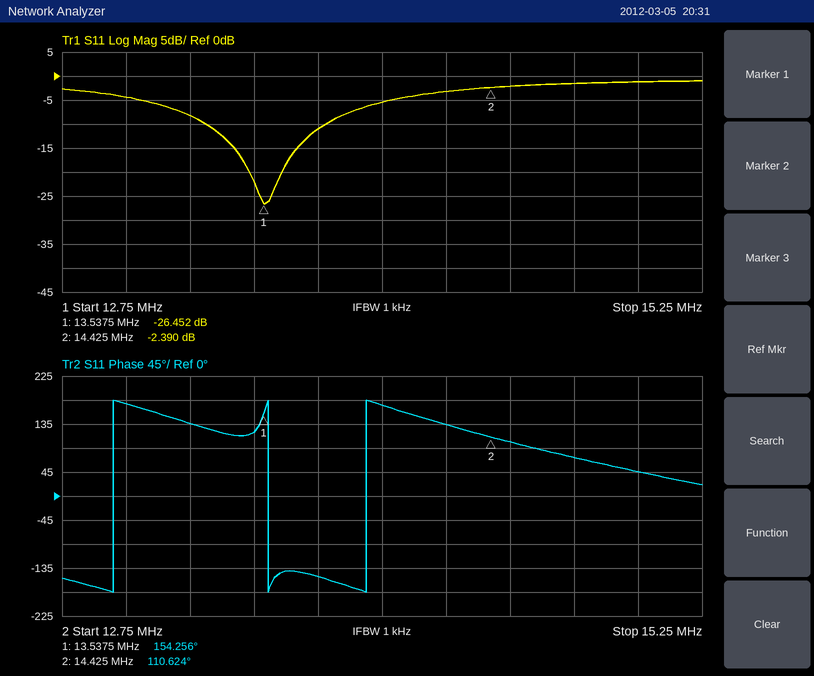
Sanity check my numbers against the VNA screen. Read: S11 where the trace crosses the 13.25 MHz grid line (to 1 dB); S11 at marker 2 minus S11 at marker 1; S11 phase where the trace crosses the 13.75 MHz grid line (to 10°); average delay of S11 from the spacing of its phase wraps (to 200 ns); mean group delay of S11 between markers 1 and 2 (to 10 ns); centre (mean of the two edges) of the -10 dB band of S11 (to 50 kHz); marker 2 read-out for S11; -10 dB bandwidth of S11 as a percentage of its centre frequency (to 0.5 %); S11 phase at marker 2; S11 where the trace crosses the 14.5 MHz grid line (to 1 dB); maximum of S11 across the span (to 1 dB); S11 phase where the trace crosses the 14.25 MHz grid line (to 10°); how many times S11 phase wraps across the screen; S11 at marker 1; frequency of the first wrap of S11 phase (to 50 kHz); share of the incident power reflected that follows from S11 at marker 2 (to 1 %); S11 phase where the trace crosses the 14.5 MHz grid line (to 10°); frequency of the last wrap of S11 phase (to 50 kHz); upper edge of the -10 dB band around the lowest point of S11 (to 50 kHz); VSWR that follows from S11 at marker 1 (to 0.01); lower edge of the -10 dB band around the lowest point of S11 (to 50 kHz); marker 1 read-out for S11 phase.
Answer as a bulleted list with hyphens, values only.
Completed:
- -8 dB
- 24.062 dB
- -150°
- 2.0 µs
- 140 ns
- 13.55 MHz
- -2.390 dB
- 3.5 %
- 110.624°
- -2 dB
- -1 dB
- 130°
- 3
- -26.452 dB
- 12.95 MHz
- 58 %
- 100°
- 13.95 MHz
- 13.80 MHz
- 1.10
- 13.30 MHz
- 154.256°
